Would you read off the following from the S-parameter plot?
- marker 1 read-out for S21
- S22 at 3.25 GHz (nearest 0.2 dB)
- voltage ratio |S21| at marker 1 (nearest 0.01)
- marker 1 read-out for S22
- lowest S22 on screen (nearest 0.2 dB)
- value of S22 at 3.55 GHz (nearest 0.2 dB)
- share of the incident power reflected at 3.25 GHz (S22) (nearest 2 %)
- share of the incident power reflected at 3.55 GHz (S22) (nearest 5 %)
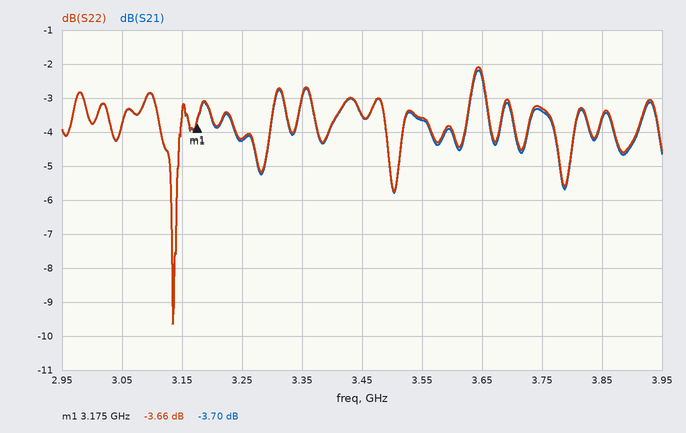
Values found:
-3.70 dB
-4.2 dB
0.65
-3.66 dB
-9.6 dB
-3.6 dB
38 %
45 %
